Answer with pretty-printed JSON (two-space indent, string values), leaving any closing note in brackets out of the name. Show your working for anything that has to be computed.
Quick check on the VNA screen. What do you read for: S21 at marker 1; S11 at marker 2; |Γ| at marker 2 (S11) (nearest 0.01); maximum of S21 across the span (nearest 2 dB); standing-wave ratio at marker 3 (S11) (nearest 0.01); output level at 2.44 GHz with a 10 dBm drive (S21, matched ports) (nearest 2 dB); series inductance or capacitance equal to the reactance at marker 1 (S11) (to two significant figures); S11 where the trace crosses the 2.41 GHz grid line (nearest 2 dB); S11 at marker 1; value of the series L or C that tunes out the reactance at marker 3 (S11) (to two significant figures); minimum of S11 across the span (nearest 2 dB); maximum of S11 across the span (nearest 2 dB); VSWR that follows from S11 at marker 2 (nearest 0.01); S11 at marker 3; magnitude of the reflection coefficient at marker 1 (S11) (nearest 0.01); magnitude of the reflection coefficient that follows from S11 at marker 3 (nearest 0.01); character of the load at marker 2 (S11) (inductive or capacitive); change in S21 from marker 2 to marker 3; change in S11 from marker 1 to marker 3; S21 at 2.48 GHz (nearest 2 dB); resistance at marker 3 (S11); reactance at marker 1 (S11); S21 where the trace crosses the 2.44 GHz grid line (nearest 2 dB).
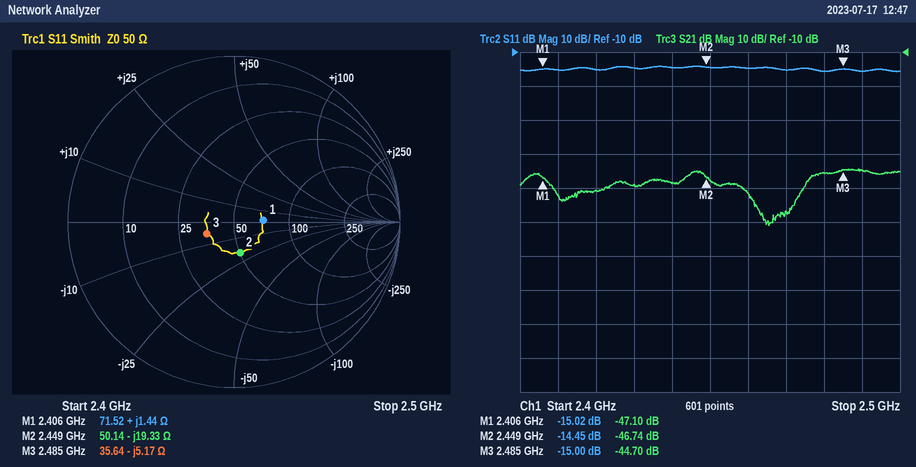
{
  "S21 at marker 1": "-47.10 dB",
  "S11 at marker 2": "-14.45 dB",
  "|Γ| at marker 2 (S11)": "0.19",
  "maximum of S21 across the span": "-44 dB",
  "standing-wave ratio at marker 3 (S11)": "1.43",
  "output level at 2.44 GHz with a 10 dBm drive (S21, matched ports)": "10 dBm + (-48 dB) = -38 dBm",
  "series inductance or capacitance equal to the reactance at marker 1 (S11)": "L = 1.44 Ω/(2π × 2.406 GHz) ≈ 95 pH",
  "S11 where the trace crosses the 2.41 GHz grid line": "-16 dB",
  "S11 at marker 1": "-15.02 dB",
  "value of the series L or C that tunes out the reactance at marker 3 (S11)": "L = 5.17 Ω/(2π × 2.485 GHz) ≈ 331 pH, so 330 pH to two significant figures",
  "minimum of S11 across the span": "-16 dB",
  "maximum of S11 across the span": "-14 dB",
  "VSWR that follows from S11 at marker 2": "(1 + 0.1895)/(1 − 0.1895) ≈ 1.47",
  "S11 at marker 3": "-15.00 dB",
  "magnitude of the reflection coefficient at marker 1 (S11)": "0.18",
  "magnitude of the reflection coefficient that follows from S11 at marker 3": "10^(-15/20) ≈ 0.18",
  "character of the load at marker 2 (S11)": "capacitive",
  "change in S21 from marker 2 to marker 3": "-44.7 − (-46.74) = 2.04 dB",
  "change in S11 from marker 1 to marker 3": "-15 − (-15.02) = 0.02 dB",
  "S21 at 2.48 GHz": "-46 dB",
  "resistance at marker 3": "35.64 Ω",
  "reactance at marker 1": "+1.44 Ω",
  "S21 where the trace crosses the 2.44 GHz grid line": "-48 dB"
}
